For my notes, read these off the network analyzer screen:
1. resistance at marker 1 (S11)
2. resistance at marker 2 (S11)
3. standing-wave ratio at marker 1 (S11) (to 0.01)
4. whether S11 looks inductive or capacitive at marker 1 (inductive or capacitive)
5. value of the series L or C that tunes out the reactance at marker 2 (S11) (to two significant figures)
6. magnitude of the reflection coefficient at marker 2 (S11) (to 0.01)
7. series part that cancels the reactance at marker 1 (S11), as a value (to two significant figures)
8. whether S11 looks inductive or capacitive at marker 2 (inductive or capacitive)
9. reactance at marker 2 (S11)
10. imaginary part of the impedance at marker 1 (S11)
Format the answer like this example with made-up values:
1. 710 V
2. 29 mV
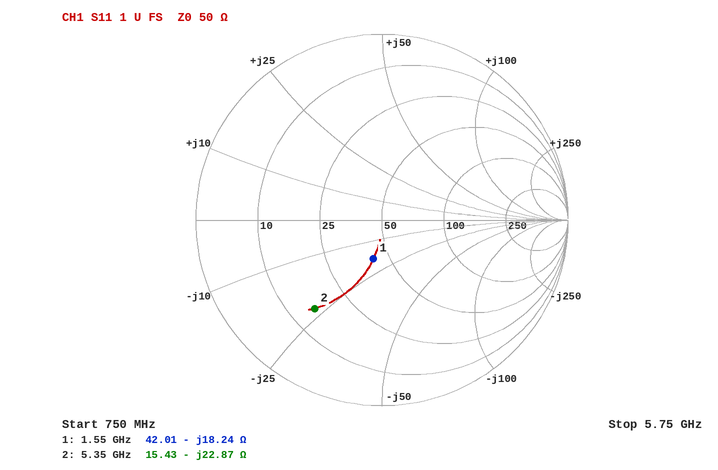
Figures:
1. 42.01 Ω
2. 15.43 Ω
3. 1.54
4. capacitive
5. 680 pH
6. 0.60
7. 1.9 nH
8. capacitive
9. -22.87 Ω
10. -18.24 Ω
